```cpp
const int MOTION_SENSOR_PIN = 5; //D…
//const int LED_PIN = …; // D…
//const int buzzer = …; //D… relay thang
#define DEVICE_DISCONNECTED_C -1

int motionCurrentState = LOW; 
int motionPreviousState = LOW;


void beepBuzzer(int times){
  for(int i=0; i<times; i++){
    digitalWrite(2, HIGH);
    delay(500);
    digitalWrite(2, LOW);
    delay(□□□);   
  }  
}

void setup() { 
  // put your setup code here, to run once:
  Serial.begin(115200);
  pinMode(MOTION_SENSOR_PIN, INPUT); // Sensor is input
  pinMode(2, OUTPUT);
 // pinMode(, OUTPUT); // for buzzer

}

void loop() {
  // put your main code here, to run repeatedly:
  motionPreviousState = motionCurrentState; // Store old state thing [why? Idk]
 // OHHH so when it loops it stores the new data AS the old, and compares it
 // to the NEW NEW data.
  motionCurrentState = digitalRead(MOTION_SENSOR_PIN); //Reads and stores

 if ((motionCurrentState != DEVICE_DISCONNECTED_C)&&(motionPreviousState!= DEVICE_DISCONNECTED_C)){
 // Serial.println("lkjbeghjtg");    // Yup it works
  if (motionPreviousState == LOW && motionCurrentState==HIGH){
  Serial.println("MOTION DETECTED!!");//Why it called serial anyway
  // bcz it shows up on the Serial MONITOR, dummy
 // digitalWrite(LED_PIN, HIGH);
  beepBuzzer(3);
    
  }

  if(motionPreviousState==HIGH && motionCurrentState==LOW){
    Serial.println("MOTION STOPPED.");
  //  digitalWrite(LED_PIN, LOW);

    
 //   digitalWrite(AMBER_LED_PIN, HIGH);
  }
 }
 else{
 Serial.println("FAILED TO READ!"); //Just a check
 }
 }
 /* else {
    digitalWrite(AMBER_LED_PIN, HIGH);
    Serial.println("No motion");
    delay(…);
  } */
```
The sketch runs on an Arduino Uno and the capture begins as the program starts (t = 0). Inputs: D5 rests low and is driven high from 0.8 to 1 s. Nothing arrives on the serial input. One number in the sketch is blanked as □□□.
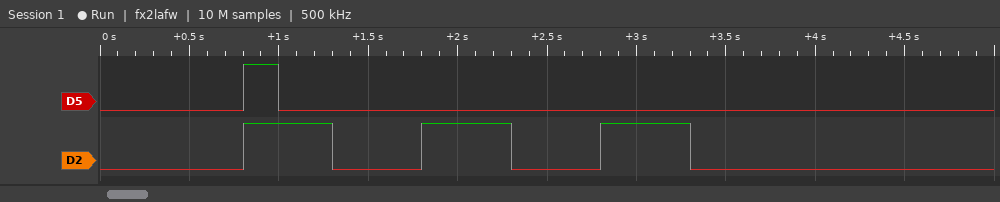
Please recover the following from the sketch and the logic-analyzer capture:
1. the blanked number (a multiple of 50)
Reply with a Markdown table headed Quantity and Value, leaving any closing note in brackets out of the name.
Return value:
| Quantity | Value |
|---|---|
| the blanked number | 500 |
